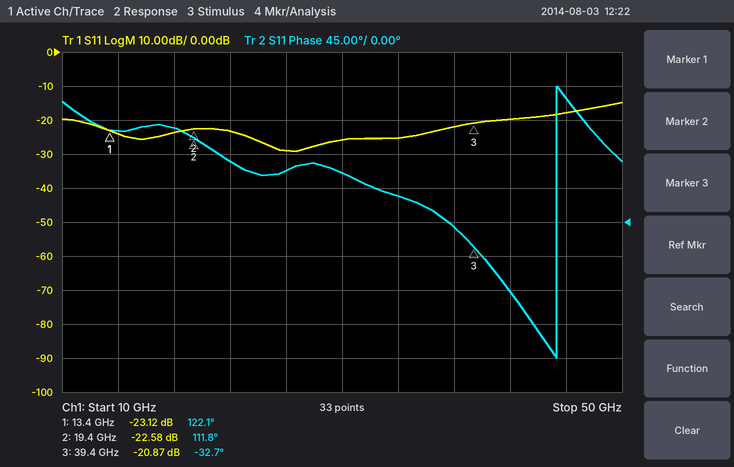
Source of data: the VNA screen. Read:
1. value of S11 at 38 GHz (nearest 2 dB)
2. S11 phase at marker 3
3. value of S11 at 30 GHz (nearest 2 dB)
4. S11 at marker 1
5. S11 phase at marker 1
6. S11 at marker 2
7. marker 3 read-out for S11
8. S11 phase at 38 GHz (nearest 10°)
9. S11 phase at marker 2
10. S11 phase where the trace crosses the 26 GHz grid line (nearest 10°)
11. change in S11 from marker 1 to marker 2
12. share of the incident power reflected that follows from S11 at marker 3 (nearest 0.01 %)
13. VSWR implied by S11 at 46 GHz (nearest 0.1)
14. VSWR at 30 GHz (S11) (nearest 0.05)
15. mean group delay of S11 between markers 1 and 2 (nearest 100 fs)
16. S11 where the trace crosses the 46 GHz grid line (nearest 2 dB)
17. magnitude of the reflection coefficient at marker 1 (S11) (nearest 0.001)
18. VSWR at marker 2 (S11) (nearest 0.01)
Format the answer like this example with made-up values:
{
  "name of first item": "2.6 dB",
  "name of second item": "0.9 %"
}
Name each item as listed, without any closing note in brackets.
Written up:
{
  "value of S11 at 38 GHz": "-22 dB",
  "S11 phase at marker 3": "-32.7°",
  "value of S11 at 30 GHz": "-26 dB",
  "S11 at marker 1": "-23.12 dB",
  "S11 phase at marker 1": "122.1°",
  "S11 at marker 2": "-22.58 dB",
  "marker 3 read-out for S11": "-20.87 dB",
  "S11 phase at 38 GHz": "-10°",
  "S11 phase at marker 2": "111.8°",
  "S11 phase where the trace crosses the 26 GHz grid line": "70°",
  "change in S11 from marker 1 to marker 2": "0.54 dB",
  "share of the incident power reflected that follows from S11 at marker 3": "0.82 %",
  "VSWR implied by S11 at 46 GHz": "1.3",
  "VSWR at 30 GHz (S11)": "1.10",
  "mean group delay of S11 between markers 1 and 2": "4.8 ps",
  "S11 where the trace crosses the 46 GHz grid line": "-18 dB",
  "magnitude of the reflection coefficient at marker 1 (S11)": "0.070",
  "VSWR at marker 2 (S11)": "1.16"
}
